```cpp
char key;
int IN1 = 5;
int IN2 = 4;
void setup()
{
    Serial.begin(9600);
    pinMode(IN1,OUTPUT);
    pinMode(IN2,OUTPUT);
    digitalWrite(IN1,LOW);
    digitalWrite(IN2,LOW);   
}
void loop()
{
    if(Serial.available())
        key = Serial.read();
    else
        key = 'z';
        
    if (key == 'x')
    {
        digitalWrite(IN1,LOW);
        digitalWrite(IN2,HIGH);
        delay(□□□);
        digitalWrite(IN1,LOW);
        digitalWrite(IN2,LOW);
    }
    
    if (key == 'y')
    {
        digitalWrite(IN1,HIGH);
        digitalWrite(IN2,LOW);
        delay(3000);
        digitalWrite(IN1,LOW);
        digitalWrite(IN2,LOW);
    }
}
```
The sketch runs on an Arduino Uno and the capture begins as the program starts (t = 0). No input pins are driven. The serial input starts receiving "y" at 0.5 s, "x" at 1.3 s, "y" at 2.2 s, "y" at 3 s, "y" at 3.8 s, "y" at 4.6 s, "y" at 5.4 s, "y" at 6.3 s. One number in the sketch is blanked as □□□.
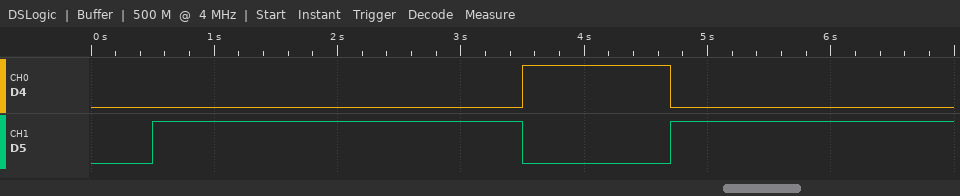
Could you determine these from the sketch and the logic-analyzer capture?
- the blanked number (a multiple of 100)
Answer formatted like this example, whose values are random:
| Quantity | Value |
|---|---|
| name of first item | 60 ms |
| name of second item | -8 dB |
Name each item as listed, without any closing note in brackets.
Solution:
| Quantity | Value |
|---|---|
| the blanked number | 1200 |
